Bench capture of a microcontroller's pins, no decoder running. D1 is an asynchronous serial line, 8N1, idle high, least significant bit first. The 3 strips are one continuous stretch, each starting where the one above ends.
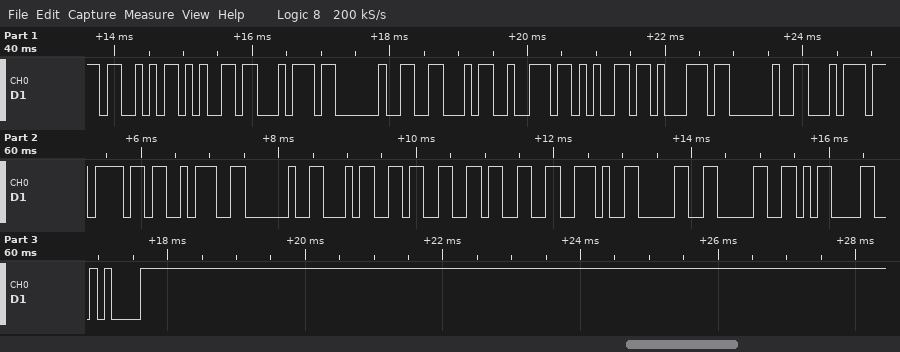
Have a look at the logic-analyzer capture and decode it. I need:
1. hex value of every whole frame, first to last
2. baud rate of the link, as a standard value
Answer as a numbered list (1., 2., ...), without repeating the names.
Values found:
1. 53 65 74 20 46 72 65 71 20 74 6F 3A 20 34 33 33 2E 30 30 0D 0A
2. 9600 baud
